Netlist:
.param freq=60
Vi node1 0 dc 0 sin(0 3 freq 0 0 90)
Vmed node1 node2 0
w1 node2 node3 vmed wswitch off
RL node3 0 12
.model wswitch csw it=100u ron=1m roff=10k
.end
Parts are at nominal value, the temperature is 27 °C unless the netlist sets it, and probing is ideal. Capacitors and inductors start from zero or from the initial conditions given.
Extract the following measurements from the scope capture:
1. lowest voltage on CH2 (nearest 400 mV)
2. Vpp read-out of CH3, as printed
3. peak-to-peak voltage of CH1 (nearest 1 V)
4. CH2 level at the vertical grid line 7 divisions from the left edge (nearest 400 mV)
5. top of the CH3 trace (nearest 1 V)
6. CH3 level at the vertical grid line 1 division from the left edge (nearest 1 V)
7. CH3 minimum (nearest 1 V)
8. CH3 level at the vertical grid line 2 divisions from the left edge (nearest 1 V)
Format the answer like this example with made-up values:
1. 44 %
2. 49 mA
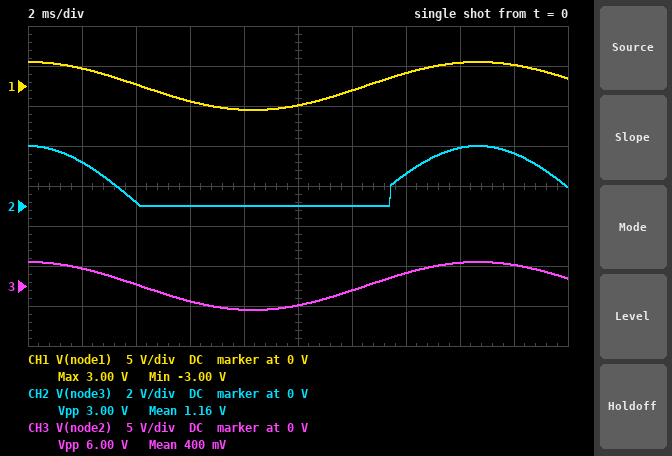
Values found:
1. 0 V
2. 6.00 V
3. 6 V
4. 1.6 V
5. 3 V
6. 2 V
7. -3 V
8. 0 V
